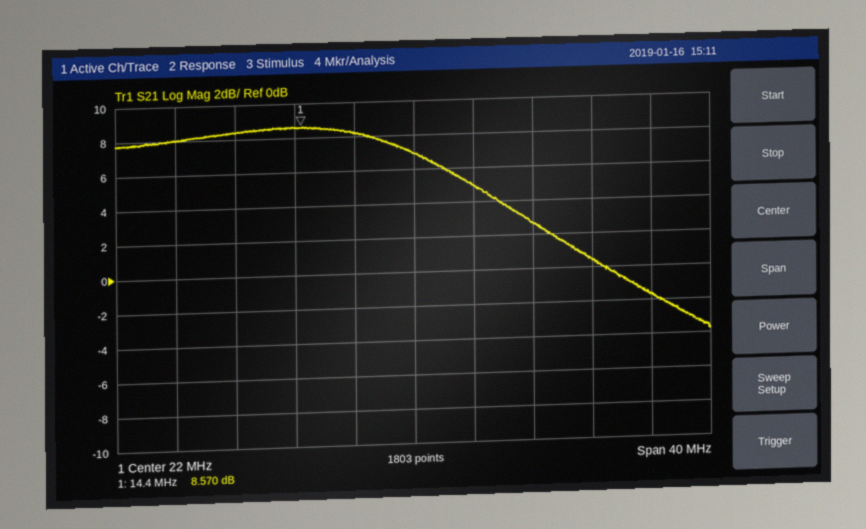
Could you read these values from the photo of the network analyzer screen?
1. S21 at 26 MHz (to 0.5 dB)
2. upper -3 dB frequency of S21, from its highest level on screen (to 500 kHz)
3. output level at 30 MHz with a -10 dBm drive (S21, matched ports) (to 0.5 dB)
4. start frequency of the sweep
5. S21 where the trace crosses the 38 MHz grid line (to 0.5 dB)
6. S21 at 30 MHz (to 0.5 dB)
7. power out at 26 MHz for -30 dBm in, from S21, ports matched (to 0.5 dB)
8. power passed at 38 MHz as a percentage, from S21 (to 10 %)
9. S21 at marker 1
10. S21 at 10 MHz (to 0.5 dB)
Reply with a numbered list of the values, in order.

1. 5.0 dB
2. 24.5 MHz
3. -7.5 dBm
4. 2 MHz
5. -1.5 dB
6. 2.5 dB
7. -25.0 dBm
8. 70 %
9. 8.570 dB
10. 8.5 dB
